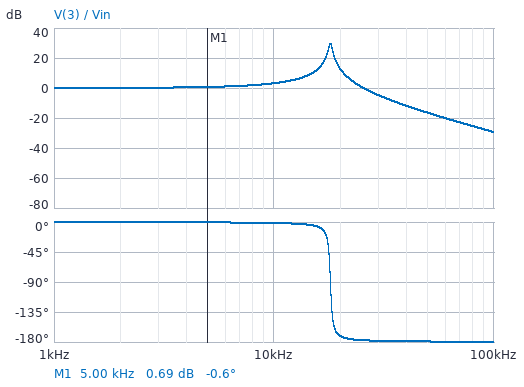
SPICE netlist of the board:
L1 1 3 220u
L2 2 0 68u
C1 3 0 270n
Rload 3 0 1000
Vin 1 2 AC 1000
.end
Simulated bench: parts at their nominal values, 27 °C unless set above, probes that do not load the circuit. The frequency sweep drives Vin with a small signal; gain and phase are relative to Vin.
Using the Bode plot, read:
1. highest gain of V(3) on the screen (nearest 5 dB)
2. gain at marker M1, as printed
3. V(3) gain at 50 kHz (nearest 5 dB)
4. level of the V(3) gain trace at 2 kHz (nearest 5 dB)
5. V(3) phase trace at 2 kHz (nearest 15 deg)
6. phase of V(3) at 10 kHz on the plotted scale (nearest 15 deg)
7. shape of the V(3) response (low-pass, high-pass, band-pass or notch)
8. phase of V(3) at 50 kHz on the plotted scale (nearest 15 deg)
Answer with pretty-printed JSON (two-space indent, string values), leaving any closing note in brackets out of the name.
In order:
{
  "highest gain of V(3) on the screen": "30 dB",
  "gain at marker M1, as printed": "0.69 dB",
  "V(3) gain at 50 kHz": "-15 dB",
  "level of the V(3) gain trace at 2 kHz": "0 dB",
  "V(3) phase trace at 2 kHz": "0 deg",
  "phase of V(3) at 10 kHz on the plotted scale": "0 deg",
  "shape of the V(3) response": "low-pass",
  "phase of V(3) at 50 kHz on the plotted scale": "-180 deg"
}
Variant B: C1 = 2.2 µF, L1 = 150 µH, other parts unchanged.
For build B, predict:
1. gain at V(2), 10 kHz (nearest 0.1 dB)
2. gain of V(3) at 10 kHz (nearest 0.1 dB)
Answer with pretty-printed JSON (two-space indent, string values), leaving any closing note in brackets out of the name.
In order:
{
  "gain at V(2), 10 kHz": "-3.6 dB",
  "gain of V(3) at 10 kHz": "1.0 dB"
}
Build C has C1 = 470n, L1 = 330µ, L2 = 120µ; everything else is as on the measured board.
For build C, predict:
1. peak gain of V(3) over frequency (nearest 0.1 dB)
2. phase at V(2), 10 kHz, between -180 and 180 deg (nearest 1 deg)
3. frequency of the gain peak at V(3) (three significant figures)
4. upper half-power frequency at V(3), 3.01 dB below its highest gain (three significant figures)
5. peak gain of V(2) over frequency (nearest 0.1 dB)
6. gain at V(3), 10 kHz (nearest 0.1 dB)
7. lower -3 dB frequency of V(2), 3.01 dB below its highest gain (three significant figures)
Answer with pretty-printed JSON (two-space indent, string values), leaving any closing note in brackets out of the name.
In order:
{
  "peak gain of V(3) over frequency": "30.2 dB",
  "phase at V(2), 10 kHz, between -180 and 180 deg": "-12 deg",
  "frequency of the gain peak at V(3)": "10.9 kHz",
  "upper half-power frequency at V(3), 3.01 dB below its highest gain": "11.1 kHz",
  "peak gain of V(2) over frequency": "18.7 dB",
  "gain at V(3), 10 kHz": "15.5 dB",
  "lower -3 dB frequency of V(2), 3.01 dB below its highest gain": "10.8 kHz"
}
